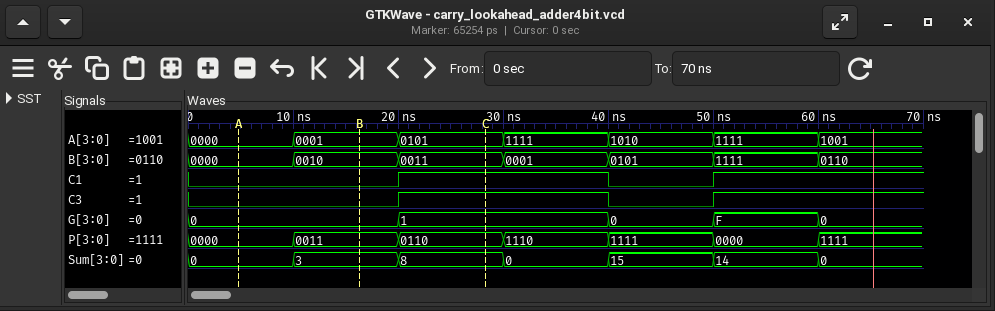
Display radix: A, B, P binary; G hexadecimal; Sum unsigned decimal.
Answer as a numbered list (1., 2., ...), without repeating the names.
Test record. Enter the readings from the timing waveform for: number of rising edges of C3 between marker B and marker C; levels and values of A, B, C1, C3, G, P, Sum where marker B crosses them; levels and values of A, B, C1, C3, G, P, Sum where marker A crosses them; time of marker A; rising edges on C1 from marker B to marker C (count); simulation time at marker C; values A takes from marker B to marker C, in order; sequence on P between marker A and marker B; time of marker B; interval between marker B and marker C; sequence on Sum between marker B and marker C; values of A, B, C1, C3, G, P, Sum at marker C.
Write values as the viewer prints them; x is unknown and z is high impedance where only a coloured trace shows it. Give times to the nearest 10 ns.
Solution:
1. 1
2. A=0001, B=0010, C1=0, C3=0, G=0, P=0011, Sum=3
3. A=0000, B=0000, C1=0, C3=0, G=0, P=0000, Sum=0
4. 0 ns
5. 1
6. 30 ns
7. 0001, 0101
8. 0000, 0011
9. 20 ns
10. 10 ns
11. 3, 8
12. A=0101, B=0011, C1=1, C3=1, G=1, P=0110, Sum=8
